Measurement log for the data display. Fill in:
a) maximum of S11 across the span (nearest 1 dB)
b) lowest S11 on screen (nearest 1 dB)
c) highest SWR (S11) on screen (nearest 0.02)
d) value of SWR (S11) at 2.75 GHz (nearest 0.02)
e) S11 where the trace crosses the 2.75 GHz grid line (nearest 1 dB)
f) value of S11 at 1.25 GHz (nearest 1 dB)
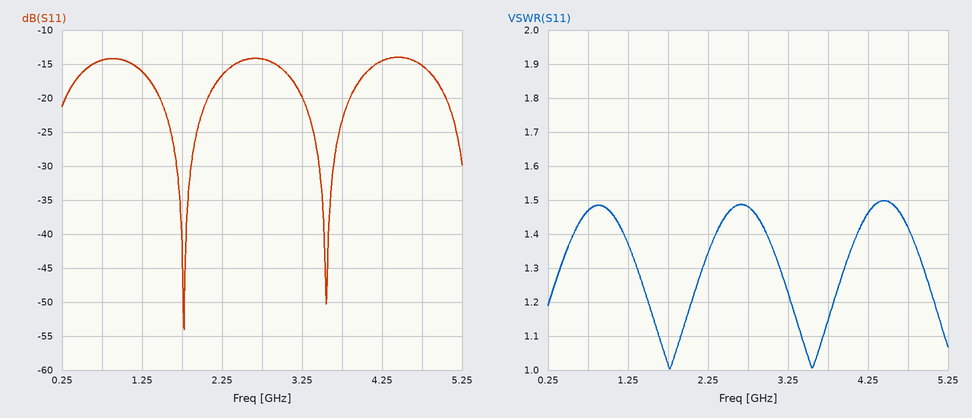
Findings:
-14 dB
-54 dB
1.50
1.48
-14 dB
-16 dB
